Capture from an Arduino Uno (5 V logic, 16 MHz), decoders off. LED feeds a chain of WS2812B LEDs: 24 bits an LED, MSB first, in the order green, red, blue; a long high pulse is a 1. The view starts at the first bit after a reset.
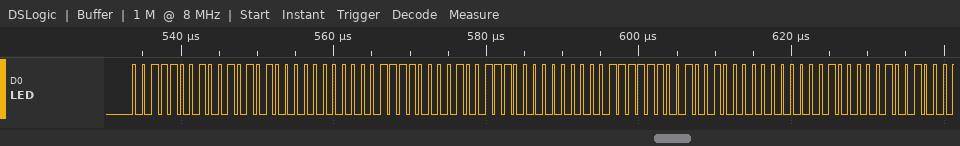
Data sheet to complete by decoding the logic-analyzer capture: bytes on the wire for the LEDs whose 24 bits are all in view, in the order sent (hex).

39 2A 00 3C 27 00 3F 24 00
